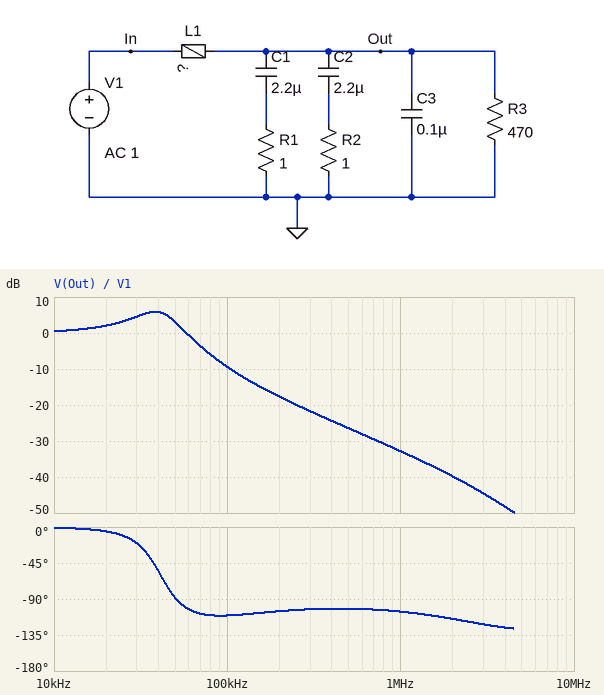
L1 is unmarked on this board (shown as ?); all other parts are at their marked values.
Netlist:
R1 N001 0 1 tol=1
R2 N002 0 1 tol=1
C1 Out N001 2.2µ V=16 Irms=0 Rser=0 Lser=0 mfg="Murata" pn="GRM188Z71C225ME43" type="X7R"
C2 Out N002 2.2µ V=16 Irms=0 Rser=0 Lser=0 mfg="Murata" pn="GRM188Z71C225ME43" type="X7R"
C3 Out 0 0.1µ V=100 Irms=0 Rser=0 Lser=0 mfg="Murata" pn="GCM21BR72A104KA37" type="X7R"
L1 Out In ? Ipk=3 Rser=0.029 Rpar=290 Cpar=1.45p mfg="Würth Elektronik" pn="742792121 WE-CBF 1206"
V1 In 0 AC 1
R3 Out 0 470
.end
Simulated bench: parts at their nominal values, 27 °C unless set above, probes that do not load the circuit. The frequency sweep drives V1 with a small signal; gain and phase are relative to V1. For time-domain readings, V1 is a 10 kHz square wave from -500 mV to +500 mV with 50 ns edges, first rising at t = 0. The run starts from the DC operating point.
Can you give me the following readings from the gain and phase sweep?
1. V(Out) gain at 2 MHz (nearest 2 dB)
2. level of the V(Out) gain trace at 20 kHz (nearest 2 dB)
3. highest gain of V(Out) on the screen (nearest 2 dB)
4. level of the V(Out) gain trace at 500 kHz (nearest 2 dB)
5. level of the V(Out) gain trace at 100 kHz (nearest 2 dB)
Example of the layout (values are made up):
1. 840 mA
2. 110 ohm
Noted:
1. -40 dB
2. 2 dB
3. 6 dB
4. -26 dB
5. -10 dB
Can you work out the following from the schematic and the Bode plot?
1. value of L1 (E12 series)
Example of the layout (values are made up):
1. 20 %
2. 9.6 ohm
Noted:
1. 3.3 µH
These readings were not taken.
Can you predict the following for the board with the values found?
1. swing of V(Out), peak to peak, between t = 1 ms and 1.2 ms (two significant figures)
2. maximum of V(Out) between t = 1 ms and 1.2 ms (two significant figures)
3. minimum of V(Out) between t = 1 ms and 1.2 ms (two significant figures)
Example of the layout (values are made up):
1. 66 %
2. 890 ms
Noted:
1. 1.9 V
2. 940 mV
3. -940 mV
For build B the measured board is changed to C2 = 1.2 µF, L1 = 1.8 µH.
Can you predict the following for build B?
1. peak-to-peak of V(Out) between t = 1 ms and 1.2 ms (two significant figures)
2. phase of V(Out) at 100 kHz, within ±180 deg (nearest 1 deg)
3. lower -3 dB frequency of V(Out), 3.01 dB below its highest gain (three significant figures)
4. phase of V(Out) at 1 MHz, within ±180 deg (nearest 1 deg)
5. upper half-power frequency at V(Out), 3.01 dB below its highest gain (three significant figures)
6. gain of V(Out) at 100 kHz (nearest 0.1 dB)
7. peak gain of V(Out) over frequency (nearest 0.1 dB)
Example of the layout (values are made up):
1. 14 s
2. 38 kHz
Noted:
1. 1.8 V
2. -96 deg
3. 28.8 kHz
4. -108 deg
5. 82.3 kHz
6. -1.5 dB
7. 4.7 dB
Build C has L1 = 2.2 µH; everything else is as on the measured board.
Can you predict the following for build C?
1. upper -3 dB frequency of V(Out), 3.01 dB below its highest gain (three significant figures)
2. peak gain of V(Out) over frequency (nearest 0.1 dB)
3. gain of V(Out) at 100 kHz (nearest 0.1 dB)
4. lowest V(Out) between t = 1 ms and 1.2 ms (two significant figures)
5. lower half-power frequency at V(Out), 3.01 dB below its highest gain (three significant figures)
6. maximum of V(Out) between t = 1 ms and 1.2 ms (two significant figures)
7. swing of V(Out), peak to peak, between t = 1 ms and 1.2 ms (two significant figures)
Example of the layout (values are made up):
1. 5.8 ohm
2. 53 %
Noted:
1. 64.0 kHz
2. 4.7 dB
3. -5.5 dB
4. -880 mV
5. 23.1 kHz
6. 880 mV
7. 1.8 V
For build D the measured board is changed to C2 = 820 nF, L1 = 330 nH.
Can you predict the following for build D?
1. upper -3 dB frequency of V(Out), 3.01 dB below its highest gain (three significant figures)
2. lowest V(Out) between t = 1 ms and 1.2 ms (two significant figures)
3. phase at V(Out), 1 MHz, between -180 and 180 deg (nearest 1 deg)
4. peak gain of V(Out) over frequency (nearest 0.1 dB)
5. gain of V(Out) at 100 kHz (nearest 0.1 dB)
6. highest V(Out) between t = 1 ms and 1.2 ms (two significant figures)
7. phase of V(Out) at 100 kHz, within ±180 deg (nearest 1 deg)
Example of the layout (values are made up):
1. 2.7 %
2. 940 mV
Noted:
1. 302 kHz
2. -680 mV
3. -100 deg
4. 1.6 dB
5. 1.4 dB
6. 680 mV
7. -14 deg
